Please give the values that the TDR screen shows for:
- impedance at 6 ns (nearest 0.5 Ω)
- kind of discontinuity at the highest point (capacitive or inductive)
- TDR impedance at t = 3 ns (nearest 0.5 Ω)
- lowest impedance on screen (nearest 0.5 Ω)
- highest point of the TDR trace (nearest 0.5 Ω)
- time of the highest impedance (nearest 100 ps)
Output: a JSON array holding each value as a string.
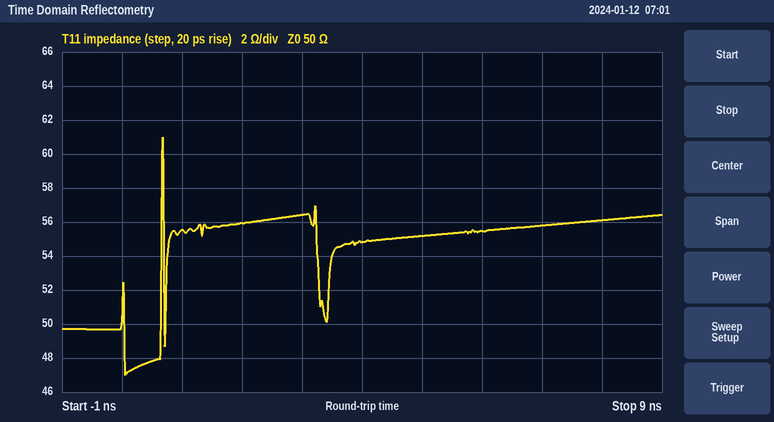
["55.5 Ω", "inductive", "56.5 Ω", "47.0 Ω", "61.0 Ω", "700 ps"]
